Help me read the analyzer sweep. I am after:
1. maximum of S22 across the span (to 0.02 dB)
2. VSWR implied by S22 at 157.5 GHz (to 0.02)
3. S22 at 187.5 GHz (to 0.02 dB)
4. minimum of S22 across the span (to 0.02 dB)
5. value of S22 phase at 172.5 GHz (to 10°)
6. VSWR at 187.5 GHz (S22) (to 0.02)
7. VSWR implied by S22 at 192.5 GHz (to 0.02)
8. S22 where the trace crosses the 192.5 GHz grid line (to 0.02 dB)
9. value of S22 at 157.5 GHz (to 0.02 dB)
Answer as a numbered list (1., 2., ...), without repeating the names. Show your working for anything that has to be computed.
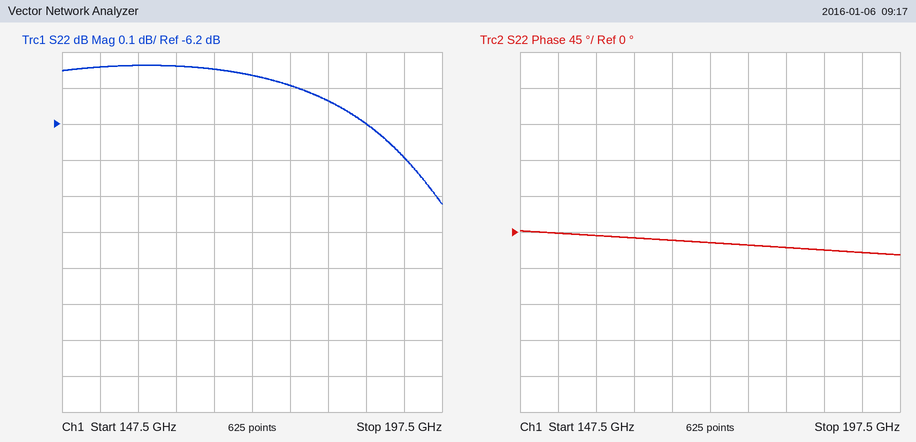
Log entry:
1. -6.04 dB
2. |Γ| = 10^(-6.04/20) = 0.4989; VSWR = (1 + 0.4989)/(1 − 0.4989) ≈ 2.99, so 3.00 to the nearest 0.02
3. -6.20 dB
4. -6.42 dB
5. -10°
6. |Γ| = 10^(-6.2/20) = 0.4898; VSWR = (1 + 0.4898)/(1 − 0.4898) ≈ 2.92
7. |Γ| = 10^(-6.3/20) = 0.4842; VSWR = (1 + 0.4842)/(1 − 0.4842) ≈ 2.88
8. -6.30 dB
9. -6.04 dB
